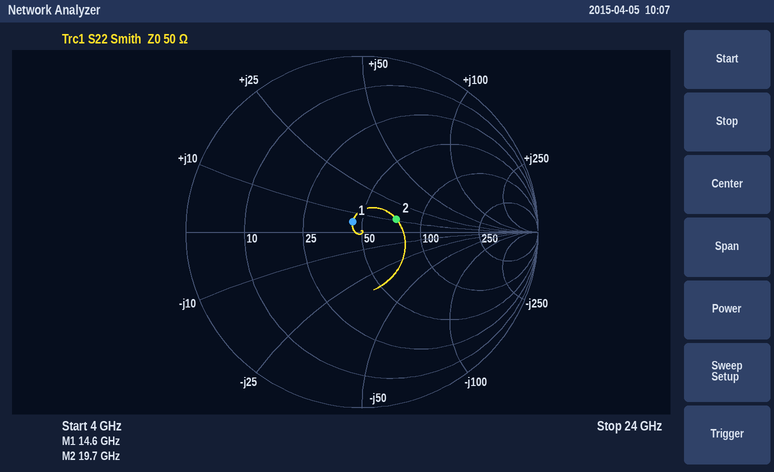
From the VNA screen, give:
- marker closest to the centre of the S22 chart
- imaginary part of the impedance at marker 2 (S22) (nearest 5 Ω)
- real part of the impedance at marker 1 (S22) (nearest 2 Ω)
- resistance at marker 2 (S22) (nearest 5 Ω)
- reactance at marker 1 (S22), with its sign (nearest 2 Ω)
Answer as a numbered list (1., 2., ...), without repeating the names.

1. marker 1
2. +10 Ω
3. 44 Ω
4. 75 Ω
5. +6 Ω
